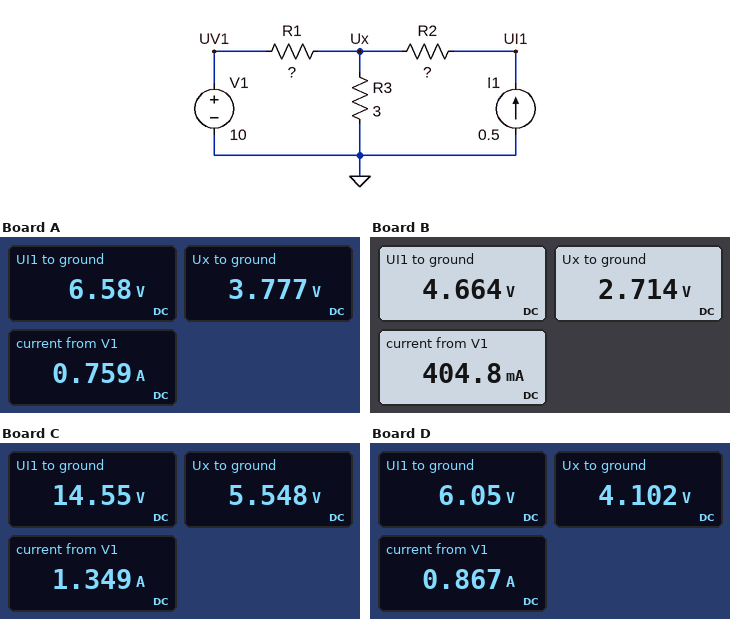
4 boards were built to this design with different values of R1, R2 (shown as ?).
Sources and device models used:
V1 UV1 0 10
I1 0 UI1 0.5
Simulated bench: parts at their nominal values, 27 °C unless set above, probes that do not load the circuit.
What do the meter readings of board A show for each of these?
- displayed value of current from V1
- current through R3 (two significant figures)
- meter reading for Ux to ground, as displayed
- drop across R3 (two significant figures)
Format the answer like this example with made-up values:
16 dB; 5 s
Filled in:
0.759 A; 1.3 A; 3.777 V; 3.8 V
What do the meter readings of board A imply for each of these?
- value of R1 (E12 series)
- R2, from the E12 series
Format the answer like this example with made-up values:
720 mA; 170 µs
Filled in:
8.2 Ω; 5.6 Ω
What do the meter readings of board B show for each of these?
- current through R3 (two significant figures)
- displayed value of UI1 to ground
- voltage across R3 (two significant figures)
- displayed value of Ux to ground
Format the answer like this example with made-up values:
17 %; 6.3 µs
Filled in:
900 mA; 4.664 V; 2.7 V; 2.714 V
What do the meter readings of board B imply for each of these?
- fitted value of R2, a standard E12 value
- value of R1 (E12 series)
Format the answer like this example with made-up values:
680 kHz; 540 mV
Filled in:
3.9 Ω; 18 Ω
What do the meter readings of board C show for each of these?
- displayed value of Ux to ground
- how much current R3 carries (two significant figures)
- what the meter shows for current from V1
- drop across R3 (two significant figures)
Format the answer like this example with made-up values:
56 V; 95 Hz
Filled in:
5.548 V; 1.8 A; 1.349 A; 5.5 V
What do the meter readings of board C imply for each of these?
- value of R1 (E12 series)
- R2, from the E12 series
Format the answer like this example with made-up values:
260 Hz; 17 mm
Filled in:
3.3 Ω; 18 Ω
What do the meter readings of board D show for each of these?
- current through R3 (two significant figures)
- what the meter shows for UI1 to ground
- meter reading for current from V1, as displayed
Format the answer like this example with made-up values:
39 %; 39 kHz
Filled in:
1.4 A; 6.05 V; 0.867 A
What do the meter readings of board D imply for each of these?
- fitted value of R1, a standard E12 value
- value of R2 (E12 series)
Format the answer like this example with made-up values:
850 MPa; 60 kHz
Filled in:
6.8 Ω; 3.9 Ω
